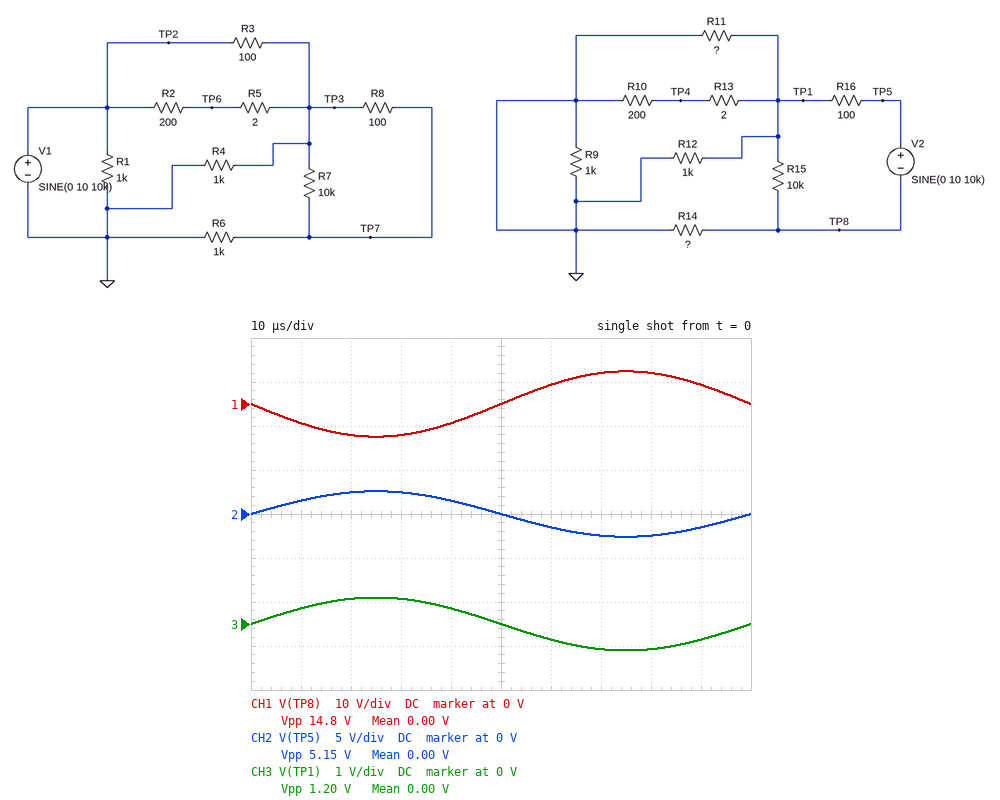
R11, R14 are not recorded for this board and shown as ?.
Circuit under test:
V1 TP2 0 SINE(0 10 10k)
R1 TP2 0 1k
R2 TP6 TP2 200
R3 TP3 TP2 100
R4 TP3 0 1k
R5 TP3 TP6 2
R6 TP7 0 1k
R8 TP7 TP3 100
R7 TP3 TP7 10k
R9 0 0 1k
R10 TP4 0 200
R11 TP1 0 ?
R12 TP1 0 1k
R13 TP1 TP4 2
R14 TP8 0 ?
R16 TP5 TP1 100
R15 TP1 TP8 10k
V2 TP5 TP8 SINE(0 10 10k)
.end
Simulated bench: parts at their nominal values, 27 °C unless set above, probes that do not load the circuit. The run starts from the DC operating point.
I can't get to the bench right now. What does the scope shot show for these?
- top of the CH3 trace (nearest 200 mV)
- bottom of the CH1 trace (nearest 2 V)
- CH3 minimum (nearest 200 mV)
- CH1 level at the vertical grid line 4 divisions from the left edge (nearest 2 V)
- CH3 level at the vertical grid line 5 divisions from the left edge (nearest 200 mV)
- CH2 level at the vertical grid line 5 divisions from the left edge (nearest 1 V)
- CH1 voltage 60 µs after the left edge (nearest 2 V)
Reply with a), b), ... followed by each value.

a) 600 mV
b) -8 V
c) -600 mV
d) -4 V
e) 0 V
f) 0 V
g) 4 V
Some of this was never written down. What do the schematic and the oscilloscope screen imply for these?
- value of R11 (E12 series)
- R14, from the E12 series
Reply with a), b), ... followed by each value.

a) 39 Ω
b) 390 Ω
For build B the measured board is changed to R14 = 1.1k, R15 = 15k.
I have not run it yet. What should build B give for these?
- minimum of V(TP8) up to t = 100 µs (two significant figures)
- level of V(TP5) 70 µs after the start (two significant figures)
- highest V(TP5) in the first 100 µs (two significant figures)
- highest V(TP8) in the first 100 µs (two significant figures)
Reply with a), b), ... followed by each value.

a) -8.9 V
b) -1.1 V
c) 1.1 V
d) 8.9 V
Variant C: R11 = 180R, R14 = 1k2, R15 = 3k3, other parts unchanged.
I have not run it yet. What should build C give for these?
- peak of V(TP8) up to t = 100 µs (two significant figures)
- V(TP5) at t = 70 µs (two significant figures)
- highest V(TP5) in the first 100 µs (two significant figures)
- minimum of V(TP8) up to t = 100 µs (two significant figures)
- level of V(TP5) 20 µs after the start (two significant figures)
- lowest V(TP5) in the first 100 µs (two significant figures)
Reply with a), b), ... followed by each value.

a) 8.4 V
b) -1.5 V
c) 1.6 V
d) -8.4 V
e) 1.5 V
f) -1.6 V
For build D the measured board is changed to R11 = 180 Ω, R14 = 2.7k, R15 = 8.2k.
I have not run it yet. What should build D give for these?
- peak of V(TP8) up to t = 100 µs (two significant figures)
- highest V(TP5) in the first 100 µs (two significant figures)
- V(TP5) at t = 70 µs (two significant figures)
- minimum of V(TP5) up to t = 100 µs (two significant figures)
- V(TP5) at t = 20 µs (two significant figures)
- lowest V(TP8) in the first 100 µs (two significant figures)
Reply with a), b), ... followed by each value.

a) 9.2 V
b) 760 mV
c) -720 mV
d) -760 mV
e) 720 mV
f) -9.2 V
